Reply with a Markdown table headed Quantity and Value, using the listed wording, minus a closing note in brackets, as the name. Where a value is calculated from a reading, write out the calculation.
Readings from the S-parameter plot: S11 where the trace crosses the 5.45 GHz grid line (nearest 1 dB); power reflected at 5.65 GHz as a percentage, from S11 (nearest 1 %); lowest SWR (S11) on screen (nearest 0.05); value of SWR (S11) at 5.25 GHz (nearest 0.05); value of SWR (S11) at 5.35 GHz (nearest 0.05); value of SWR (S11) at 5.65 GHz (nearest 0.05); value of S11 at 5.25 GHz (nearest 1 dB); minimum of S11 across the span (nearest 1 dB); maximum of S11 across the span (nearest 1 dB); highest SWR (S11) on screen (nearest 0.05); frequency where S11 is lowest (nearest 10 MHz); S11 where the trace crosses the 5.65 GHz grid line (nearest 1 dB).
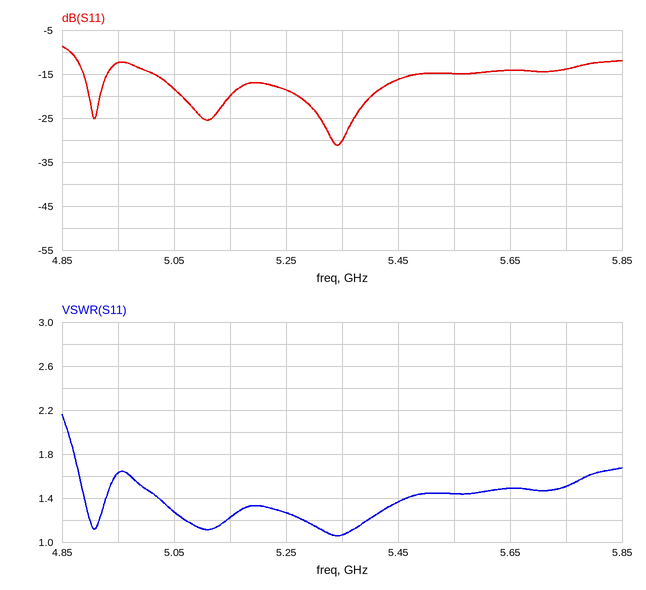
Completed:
| Quantity | Value |
|---|---|
| S11 where the trace crosses the 5.45 GHz grid line | -16 dB |
| power reflected at 5.65 GHz as a percentage, from S11 | 10^(-14/10) ≈ 4 % |
| lowest SWR (S11) on screen | 1.05 |
| value of SWR (S11) at 5.25 GHz | 1.25 |
| value of SWR (S11) at 5.35 GHz | 1.05 |
| value of SWR (S11) at 5.65 GHz | 1.50 |
| value of S11 at 5.25 GHz | -19 dB |
| minimum of S11 across the span | -31 dB |
| maximum of S11 across the span | -9 dB |
| highest SWR (S11) on screen | 2.15 |
| frequency where S11 is lowest | 5.34 GHz |
| S11 where the trace crosses the 5.65 GHz grid line | -14 dB |
